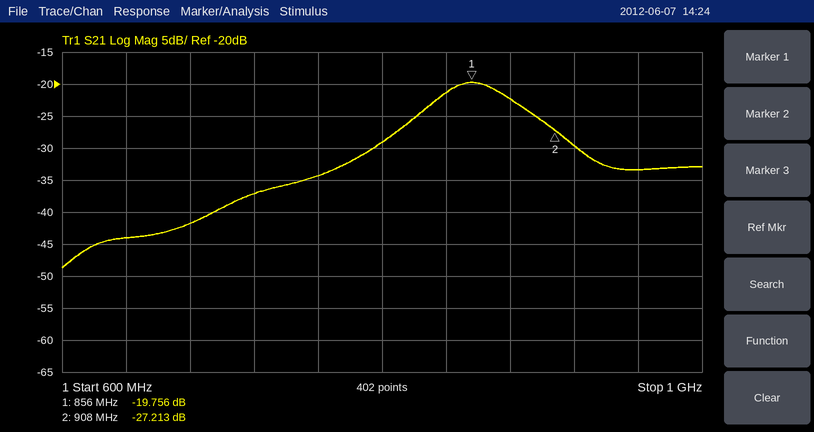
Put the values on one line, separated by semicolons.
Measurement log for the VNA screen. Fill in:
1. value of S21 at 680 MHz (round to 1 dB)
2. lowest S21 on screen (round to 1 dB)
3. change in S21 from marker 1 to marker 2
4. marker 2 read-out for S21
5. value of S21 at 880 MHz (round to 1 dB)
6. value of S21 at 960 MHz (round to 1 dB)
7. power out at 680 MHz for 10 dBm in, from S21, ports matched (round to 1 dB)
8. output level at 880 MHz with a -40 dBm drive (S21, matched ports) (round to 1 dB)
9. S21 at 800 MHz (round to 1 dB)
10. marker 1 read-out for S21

-42 dB; -49 dB; -7.457 dB; -27.213 dB; -22 dB; -33 dB; -32 dBm; -62 dBm; -29 dB; -19.756 dB
